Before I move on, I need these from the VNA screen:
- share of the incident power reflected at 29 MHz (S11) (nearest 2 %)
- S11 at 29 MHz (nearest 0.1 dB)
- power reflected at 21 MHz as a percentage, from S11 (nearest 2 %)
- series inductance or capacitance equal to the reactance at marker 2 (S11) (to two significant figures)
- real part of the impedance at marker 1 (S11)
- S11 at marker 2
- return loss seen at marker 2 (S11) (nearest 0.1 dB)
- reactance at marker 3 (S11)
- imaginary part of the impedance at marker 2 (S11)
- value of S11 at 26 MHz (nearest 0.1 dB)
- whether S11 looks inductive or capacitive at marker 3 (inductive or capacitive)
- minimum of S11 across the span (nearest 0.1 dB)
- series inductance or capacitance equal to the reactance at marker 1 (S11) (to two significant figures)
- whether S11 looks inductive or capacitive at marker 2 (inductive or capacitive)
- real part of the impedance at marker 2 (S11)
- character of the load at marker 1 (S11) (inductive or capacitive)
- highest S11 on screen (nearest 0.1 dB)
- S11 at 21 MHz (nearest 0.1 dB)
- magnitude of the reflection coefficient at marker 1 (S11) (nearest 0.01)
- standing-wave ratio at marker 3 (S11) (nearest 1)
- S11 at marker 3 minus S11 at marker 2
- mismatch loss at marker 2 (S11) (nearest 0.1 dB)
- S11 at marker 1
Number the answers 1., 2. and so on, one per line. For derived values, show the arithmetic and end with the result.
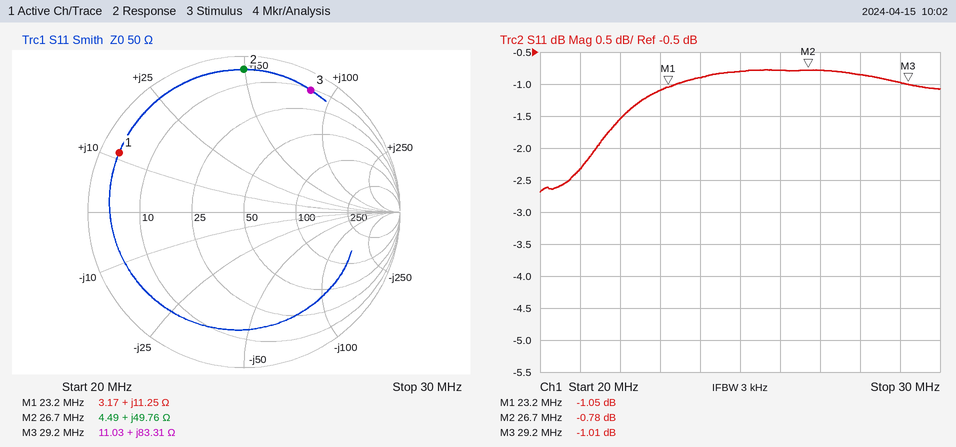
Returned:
1. 10^(-1/10) ≈ 79.4 %, so 80 % to the nearest 2 %
2. -1.0 dB
3. 10^(-2.3/10) ≈ 58.9 %, so 58 % to the nearest 2 %
4. L = 49.76 Ω/(2π × 26.7 MHz) ≈ 297 nH, so 300 nH to two significant figures
5. 3.17 Ω
6. -0.78 dB
7. 0.8 dB
8. +83.31 Ω
9. +49.76 Ω
10. -0.8 dB
11. inductive
12. -2.7 dB
13. L = 11.25 Ω/(2π × 23.2 MHz) ≈ 77 nH
14. inductive
15. 4.49 Ω
16. inductive
17. -0.8 dB
18. -2.3 dB
19. 0.89
20. 17
21. -1.01 − (-0.78) = -0.23 dB
22. −10 log10(1 − 10^(-0.78/10)) ≈ 7.8 dB
23. -1.05 dB
